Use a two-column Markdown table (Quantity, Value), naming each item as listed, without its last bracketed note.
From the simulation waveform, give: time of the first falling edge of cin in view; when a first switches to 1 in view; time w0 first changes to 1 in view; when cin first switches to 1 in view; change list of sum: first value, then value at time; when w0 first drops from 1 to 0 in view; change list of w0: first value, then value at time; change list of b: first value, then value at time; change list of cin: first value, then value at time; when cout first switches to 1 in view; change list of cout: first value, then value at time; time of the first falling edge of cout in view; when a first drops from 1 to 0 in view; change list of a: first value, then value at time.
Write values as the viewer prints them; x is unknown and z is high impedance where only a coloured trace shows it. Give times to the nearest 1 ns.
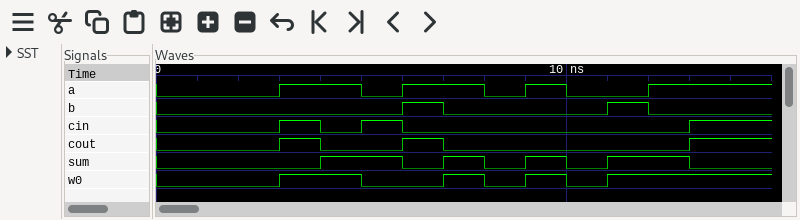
| Quantity | Value |
|---|---|
| time of the first falling edge of cin in view | 4 ns |
| when a first switches to 1 in view | 3 ns |
| time w0 first changes to 1 in view | 3 ns |
| when cin first switches to 1 in view | 3 ns |
| change list of sum: first value, then value at time | 0, 1 at 4 ns, 0 at 6 ns, 1 at 7 ns, 0 at 8 ns, 1 at 9 ns, 0 at 10 ns, 1 at 11 ns, 0 at 13 ns |
| when w0 first drops from 1 to 0 in view | 5 ns |
| change list of w0: first value, then value at time | 0, 1 at 3 ns, 0 at 5 ns, 1 at 7 ns, 0 at 8 ns, 1 at 9 ns, 0 at 10 ns, 1 at 11 ns |
| change list of b: first value, then value at time | 0, 1 at 6 ns, 0 at 7 ns, 1 at 11 ns, 0 at 12 ns |
| change list of cin: first value, then value at time | 0, 1 at 3 ns, 0 at 4 ns, 1 at 5 ns, 0 at 6 ns, 1 at 13 ns |
| when cout first switches to 1 in view | 3 ns |
| change list of cout: first value, then value at time | 0, 1 at 3 ns, 0 at 4 ns, 1 at 6 ns, 0 at 7 ns, 1 at 13 ns |
| time of the first falling edge of cout in view | 4 ns |
| when a first drops from 1 to 0 in view | 5 ns |
| change list of a: first value, then value at time | 0, 1 at 3 ns, 0 at 5 ns, 1 at 6 ns, 0 at 8 ns, 1 at 9 ns, 0 at 10 ns, 1 at 12 ns |
